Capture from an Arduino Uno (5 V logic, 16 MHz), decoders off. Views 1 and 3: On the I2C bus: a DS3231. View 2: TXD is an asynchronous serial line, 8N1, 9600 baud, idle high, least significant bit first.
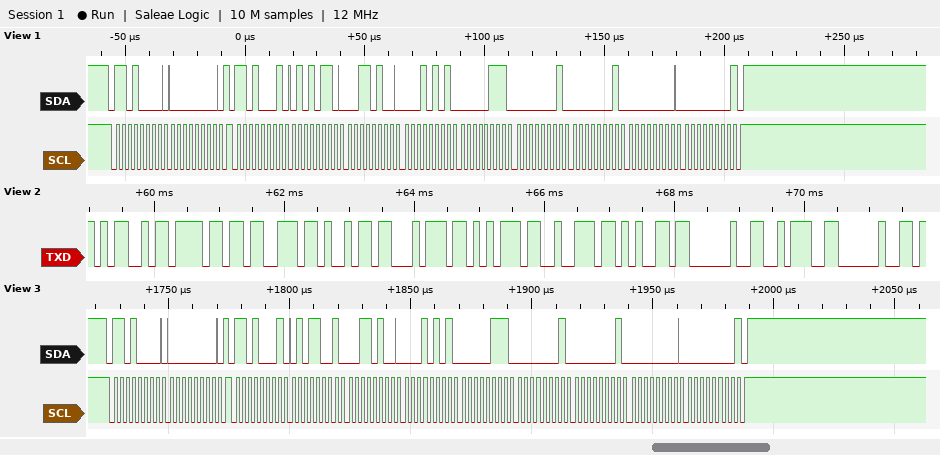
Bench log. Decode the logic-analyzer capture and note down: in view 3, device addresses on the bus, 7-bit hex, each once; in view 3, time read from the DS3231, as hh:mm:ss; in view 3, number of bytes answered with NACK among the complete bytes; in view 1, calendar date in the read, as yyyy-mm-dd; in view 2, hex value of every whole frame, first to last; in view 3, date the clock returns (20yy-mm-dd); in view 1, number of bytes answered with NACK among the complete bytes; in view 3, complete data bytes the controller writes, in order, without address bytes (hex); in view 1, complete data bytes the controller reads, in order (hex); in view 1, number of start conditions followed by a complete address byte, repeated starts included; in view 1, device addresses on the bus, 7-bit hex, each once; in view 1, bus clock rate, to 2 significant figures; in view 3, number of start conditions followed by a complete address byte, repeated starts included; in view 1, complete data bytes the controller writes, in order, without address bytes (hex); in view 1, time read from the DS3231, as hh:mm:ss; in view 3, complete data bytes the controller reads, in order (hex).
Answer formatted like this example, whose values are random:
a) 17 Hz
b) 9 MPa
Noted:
a) 0x68
b) 15:34:59
c) 1
d) 2000-01-01
e) 0x4D 0x6F 0x73 0x69 0x74 0x75 0x72 0x65 0x20 0x3A 0x20
f) 2000-01-01
g) 1
h) 00
i) 56 34 15 07 01 01 00 00
j) 2
k) 0x68
l) 400 kHz
m) 2
n) 00
o) 15:34:56
p) 59 34 15 07 01 01 00 00
